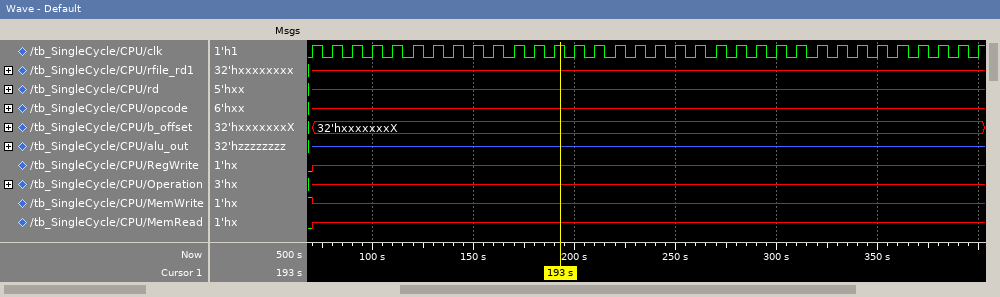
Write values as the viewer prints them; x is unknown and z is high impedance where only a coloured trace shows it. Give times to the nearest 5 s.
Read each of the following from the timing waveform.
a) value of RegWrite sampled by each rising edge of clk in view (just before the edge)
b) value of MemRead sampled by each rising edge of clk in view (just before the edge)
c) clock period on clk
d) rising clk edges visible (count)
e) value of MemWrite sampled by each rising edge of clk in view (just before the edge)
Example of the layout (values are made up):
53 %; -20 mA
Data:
0 x x x x x x x x x x x x x x x x x x x x x x x x x x x x x x x x x; 0 x x x x x x x x x x x x x x x x x x x x x x x x x x x x x x x x x; 10 s; 34; 1 x x x x x x x x x x x x x x x x x x x x x x x x x x x x x x x x x
